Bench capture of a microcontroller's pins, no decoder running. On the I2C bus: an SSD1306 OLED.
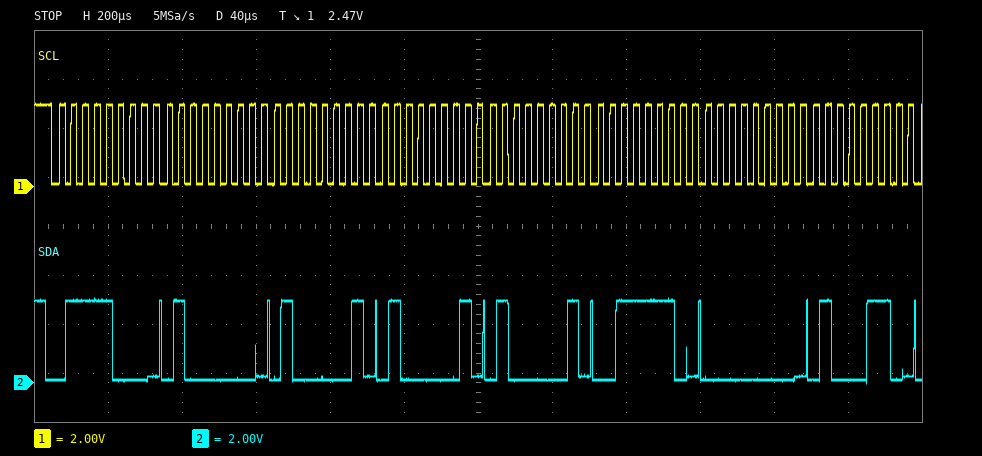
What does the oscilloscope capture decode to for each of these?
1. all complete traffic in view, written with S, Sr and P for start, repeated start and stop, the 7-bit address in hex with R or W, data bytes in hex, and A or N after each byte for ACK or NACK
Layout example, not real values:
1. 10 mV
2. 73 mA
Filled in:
1. S 3CW A 40 A 41 A 41 A 41 A 3E A 00 A 46 A
